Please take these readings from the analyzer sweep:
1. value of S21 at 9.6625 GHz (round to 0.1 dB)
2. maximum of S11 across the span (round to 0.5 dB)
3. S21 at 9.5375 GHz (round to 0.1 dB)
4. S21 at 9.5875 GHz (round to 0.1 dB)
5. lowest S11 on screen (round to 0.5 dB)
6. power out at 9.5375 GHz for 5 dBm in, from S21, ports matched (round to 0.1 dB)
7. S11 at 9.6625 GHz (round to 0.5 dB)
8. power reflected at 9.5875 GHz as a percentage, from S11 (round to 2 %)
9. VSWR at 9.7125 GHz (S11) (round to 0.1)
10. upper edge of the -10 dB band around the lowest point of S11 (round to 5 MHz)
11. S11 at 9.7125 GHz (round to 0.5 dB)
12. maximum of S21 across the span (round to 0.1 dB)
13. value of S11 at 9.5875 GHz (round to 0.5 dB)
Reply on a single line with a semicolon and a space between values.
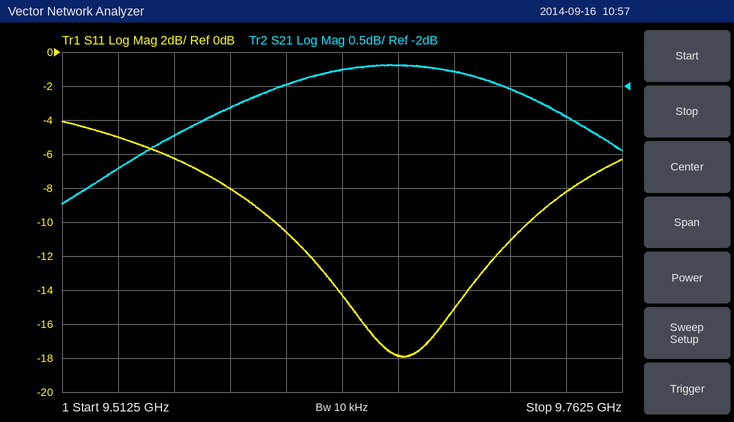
-1.7 dB; -4.0 dB; -3.2 dB; -2.3 dB; -18.0 dB; 1.8 dBm; -18.0 dB; 16 %; 1.8; 9.720 GHz; -11.0 dB; -1.7 dB; -8.0 dB
